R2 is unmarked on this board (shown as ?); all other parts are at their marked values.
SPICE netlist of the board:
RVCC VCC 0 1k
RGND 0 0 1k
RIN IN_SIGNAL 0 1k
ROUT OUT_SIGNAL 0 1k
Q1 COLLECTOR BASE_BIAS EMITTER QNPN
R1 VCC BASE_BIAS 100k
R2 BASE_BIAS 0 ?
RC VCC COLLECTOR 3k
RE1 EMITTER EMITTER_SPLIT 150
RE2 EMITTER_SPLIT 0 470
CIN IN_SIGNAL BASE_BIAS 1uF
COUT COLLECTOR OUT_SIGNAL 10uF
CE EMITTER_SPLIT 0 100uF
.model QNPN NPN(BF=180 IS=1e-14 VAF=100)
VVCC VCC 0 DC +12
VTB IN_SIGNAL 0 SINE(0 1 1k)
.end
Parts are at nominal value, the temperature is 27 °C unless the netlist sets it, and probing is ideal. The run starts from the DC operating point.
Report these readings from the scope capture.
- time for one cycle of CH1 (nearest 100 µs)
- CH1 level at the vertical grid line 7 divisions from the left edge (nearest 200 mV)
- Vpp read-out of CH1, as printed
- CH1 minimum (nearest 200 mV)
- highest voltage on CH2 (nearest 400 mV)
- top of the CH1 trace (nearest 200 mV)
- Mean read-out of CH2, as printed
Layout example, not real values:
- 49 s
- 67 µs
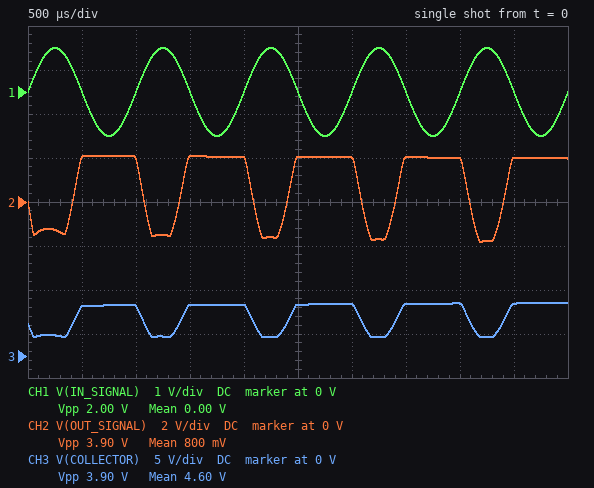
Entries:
- 1.0 ms
- 0 V
- 2.00 V
- -1.0 V
- 2.0 V
- 1.0 V
- 800 mV
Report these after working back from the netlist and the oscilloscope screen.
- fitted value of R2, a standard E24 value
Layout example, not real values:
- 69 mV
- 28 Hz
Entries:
- 30 kΩ
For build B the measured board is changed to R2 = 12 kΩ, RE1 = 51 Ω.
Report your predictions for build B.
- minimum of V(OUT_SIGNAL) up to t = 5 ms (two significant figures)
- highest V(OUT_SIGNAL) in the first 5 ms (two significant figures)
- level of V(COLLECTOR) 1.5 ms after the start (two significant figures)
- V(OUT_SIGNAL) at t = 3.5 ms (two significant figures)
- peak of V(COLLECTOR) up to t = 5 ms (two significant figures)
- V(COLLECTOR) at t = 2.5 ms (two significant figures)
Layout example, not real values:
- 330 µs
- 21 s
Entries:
- -7.5 V
- 990 mV
- 9.3 V
- 960 mV
- 9.4 V
- 9.2 V
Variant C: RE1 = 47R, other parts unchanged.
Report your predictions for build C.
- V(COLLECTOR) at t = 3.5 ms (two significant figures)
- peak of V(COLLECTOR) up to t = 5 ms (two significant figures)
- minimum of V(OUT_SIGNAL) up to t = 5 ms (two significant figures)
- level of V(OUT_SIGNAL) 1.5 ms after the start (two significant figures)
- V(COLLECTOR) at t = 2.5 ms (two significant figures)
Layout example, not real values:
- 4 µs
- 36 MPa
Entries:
- 5.2 V
- 5.4 V
- -1.3 V
- 2.4 V
- 5.0 V
